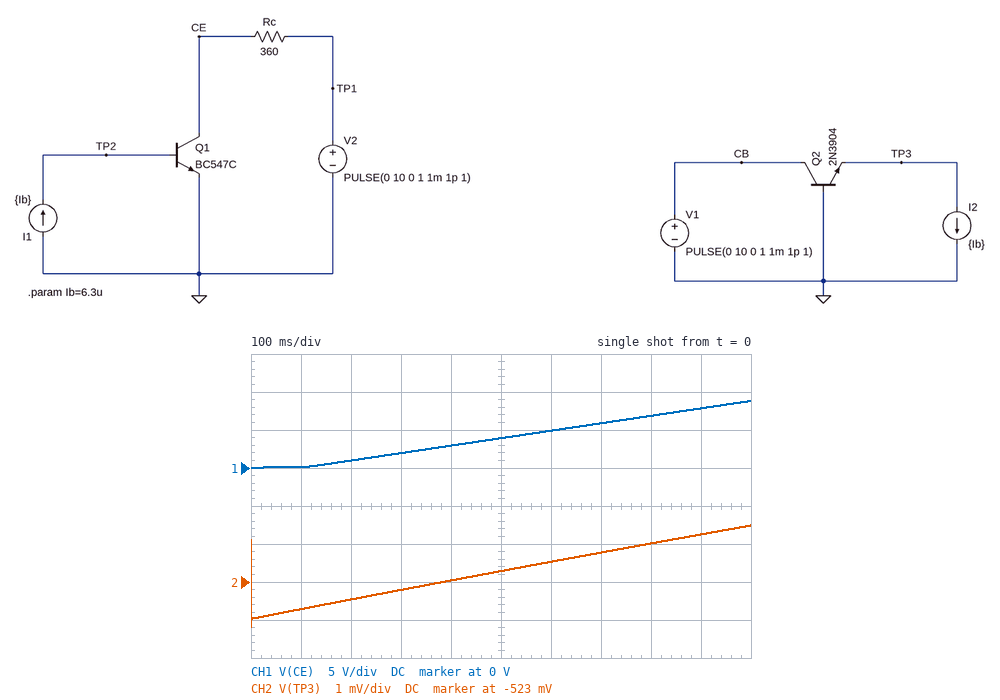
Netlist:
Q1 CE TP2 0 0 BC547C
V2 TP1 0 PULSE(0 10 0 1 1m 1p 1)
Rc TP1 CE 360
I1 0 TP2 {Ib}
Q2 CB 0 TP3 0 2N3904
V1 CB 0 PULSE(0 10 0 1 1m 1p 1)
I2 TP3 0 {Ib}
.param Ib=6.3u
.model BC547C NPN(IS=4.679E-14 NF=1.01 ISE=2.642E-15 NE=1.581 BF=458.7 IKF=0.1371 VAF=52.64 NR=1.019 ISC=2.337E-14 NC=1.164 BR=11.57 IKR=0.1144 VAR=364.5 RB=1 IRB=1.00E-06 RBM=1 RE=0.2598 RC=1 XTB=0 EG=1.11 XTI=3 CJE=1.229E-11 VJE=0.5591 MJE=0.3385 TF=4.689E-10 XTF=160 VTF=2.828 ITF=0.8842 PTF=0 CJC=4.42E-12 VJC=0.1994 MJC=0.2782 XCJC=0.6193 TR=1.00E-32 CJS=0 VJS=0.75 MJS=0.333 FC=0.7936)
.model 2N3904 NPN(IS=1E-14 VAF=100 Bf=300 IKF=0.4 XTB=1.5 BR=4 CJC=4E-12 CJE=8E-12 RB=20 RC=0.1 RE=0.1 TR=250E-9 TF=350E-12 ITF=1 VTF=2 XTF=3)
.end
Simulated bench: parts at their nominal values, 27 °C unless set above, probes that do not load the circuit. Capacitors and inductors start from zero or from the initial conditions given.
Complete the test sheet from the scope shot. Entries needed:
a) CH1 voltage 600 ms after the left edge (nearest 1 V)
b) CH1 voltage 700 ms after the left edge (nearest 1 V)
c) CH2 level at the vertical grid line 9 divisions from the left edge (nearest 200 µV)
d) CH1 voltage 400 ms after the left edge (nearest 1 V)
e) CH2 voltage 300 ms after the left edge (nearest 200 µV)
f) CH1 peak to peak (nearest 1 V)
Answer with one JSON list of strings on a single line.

["5 V", "6 V", "-521.8 mV", "3 V", "-523.2 mV", "9 V"]
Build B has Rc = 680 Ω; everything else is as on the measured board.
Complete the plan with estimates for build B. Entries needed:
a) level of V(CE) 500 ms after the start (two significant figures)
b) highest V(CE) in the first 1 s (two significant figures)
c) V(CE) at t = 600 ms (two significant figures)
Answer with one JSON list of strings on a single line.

["3.0 V", "7.8 V", "4.0 V"]
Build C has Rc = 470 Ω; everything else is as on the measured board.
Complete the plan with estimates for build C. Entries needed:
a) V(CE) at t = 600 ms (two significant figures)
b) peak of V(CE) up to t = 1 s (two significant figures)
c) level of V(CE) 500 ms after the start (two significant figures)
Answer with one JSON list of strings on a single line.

["4.6 V", "8.5 V", "3.6 V"]
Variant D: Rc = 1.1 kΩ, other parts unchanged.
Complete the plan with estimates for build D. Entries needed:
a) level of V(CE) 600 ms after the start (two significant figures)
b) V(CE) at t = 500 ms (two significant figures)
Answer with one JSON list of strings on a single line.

["2.8 V", "1.8 V"]
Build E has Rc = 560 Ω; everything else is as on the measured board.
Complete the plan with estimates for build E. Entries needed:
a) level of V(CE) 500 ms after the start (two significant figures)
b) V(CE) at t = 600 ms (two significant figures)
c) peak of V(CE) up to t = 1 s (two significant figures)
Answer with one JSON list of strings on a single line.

["3.3 V", "4.3 V", "8.2 V"]
